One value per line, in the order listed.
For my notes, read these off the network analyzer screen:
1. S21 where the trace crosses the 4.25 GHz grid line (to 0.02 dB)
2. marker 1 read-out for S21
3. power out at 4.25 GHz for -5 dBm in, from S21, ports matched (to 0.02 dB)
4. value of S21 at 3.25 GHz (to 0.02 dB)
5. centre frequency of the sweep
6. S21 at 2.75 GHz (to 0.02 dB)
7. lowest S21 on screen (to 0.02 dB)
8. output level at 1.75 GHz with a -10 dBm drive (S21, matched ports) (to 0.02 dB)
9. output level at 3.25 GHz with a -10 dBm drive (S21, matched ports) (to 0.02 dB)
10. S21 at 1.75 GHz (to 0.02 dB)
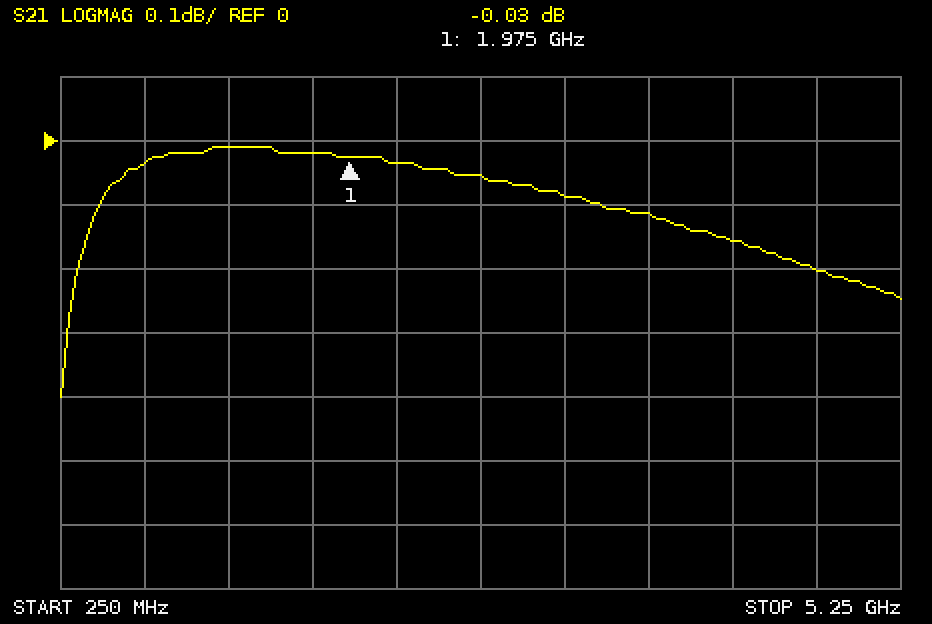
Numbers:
-0.16 dB
-0.03 dB
-5.16 dBm
-0.08 dB
2.75 GHz
-0.06 dB
-0.40 dB
-10.02 dBm
-10.08 dBm
-0.02 dB
